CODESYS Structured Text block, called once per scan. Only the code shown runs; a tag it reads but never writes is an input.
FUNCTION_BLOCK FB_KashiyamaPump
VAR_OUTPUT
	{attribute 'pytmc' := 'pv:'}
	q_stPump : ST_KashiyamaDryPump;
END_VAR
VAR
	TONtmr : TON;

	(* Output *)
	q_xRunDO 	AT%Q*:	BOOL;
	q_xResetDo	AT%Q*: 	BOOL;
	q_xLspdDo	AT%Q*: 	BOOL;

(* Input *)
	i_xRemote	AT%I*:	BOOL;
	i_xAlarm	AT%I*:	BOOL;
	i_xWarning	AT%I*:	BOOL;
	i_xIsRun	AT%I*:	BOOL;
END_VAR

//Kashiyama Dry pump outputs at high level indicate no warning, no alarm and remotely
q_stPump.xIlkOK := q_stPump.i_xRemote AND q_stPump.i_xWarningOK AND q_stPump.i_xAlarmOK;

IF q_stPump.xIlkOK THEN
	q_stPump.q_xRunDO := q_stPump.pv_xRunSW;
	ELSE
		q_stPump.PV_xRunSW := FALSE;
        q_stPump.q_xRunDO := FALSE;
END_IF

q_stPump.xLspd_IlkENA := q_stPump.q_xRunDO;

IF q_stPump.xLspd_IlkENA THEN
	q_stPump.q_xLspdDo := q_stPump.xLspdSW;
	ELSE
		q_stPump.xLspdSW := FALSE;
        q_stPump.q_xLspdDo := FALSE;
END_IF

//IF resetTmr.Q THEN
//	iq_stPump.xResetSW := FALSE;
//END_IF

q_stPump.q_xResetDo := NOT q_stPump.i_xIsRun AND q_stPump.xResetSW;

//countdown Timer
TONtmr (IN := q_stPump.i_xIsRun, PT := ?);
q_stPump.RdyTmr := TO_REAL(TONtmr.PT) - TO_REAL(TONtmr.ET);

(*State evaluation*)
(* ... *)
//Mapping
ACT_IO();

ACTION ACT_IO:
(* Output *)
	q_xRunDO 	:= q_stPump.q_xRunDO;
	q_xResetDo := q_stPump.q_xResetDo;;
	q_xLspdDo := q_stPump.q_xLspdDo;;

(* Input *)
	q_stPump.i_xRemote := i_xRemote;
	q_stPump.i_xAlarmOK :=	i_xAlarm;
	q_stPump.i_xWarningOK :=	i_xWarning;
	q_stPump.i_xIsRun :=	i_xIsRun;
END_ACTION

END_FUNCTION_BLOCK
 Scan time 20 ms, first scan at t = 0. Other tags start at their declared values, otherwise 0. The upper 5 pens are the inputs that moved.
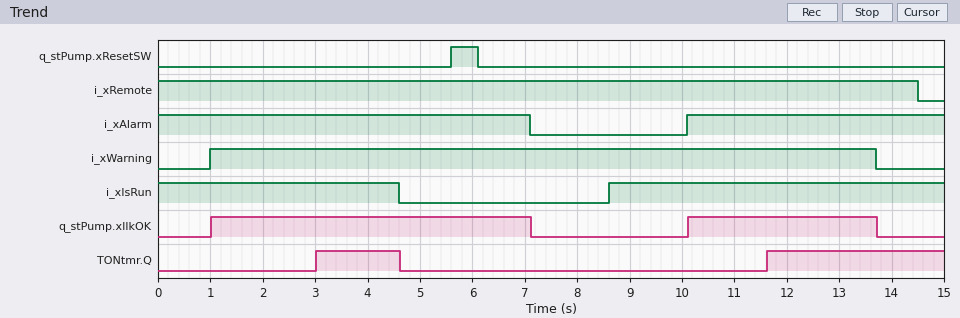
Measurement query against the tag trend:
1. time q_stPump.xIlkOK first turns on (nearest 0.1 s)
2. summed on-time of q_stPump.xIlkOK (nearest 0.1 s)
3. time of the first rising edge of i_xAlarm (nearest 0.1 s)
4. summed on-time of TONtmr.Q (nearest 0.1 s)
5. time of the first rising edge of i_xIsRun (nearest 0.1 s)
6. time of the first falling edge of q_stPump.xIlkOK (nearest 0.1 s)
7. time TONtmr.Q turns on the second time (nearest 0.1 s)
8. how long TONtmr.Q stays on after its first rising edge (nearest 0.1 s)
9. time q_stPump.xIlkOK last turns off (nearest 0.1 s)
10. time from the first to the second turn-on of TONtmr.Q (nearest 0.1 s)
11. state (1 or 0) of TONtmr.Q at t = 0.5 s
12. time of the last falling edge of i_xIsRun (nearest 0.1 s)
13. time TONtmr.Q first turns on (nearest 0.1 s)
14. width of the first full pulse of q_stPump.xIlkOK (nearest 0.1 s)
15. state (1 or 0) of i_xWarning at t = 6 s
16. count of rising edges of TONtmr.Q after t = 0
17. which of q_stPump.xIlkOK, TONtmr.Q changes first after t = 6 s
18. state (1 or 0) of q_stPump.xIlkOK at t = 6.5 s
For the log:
1.0 s
9.7 s
10.1 s
5.0 s
8.6 s
7.1 s
11.6 s
1.6 s
13.7 s
8.6 s
0
4.6 s
3.0 s
6.1 s
1
2
q_stPump.xIlkOK
1
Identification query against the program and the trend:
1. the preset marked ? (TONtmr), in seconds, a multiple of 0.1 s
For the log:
3.0 s
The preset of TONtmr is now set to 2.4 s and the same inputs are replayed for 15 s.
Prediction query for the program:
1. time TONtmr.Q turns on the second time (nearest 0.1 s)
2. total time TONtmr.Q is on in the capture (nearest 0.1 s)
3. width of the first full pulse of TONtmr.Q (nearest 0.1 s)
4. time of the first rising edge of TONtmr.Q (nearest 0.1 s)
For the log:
11.0 s
6.2 s
2.2 s
2.4 s
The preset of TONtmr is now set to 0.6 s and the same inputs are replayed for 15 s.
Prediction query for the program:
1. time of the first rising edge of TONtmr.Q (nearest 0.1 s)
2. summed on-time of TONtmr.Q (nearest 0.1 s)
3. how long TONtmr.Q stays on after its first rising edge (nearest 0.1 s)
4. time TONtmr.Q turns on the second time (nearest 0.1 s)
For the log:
0.6 s
9.8 s
4.0 s
9.2 s
